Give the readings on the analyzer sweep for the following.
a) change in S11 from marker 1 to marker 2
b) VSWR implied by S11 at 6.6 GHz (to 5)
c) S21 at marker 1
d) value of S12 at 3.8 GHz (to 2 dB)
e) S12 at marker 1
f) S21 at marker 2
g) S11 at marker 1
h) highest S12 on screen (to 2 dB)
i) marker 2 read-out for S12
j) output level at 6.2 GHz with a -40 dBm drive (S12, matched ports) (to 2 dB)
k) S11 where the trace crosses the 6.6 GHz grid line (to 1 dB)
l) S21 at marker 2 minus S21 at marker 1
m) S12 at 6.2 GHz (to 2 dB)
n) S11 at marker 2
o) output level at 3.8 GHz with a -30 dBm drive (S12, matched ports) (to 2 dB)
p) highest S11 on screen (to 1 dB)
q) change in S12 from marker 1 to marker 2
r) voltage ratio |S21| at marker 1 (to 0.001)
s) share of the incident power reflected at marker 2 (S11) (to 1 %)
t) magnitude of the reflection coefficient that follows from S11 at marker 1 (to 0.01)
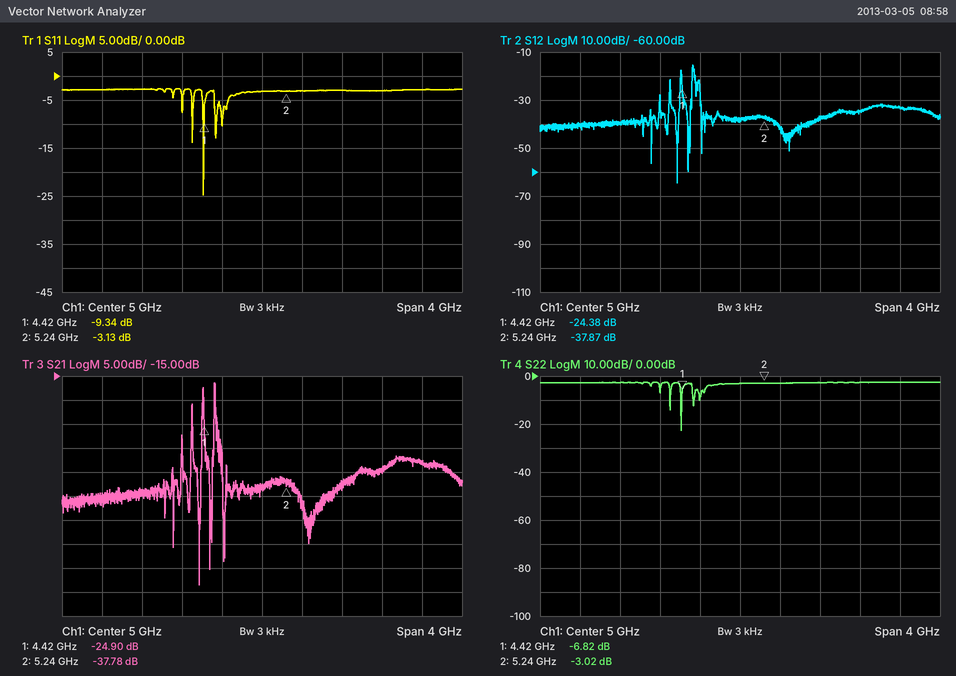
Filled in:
6.21 dB
5
-24.90 dB
-40 dB
-24.38 dB
-37.78 dB
-9.34 dB
-16 dB
-37.87 dB
-74 dBm
-3 dB
-12.88 dB
-34 dB
-3.13 dB
-70 dBm
-3 dB
-13.49 dB
0.057
49 %
0.34
